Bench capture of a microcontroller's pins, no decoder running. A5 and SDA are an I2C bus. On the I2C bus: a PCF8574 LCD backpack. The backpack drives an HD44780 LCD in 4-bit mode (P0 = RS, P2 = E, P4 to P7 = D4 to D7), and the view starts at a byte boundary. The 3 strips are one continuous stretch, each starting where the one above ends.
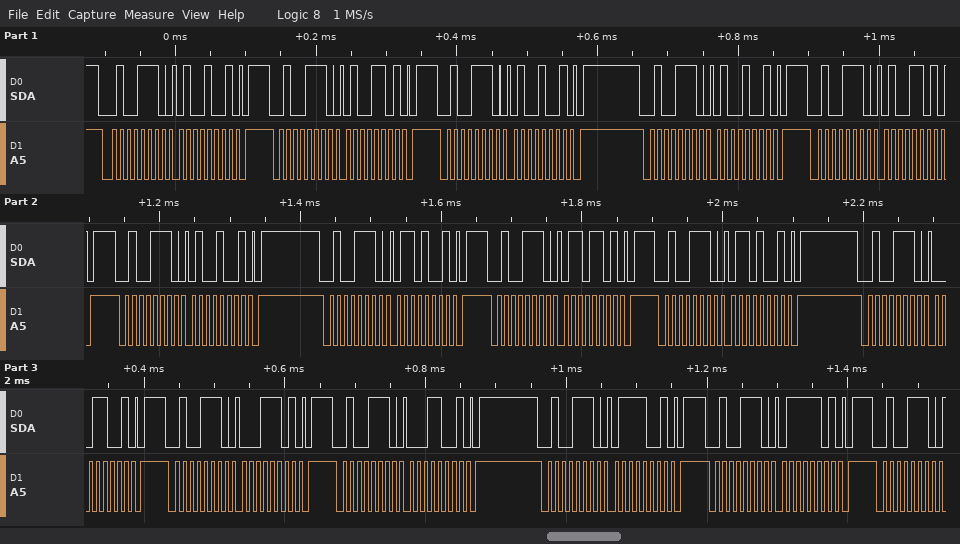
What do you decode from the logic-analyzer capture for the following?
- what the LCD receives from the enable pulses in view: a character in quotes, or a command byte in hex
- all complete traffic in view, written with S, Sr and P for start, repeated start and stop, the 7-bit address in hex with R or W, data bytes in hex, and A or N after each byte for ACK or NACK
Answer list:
'D' 'a'
S 27W A 49 A P S 27W A 4D A P S 27W A 49 A P S 27W A 49 A P S 27W A 4D A P S 27W A 49 A P S 27W A 69 A P S 27W A 6D A P S 27W A 69 A P S 27W A 19 A P S 27W A 1D A P S 27W A 19 A P S 27W A 79 A P S 27W A 7D A P S 27W A
